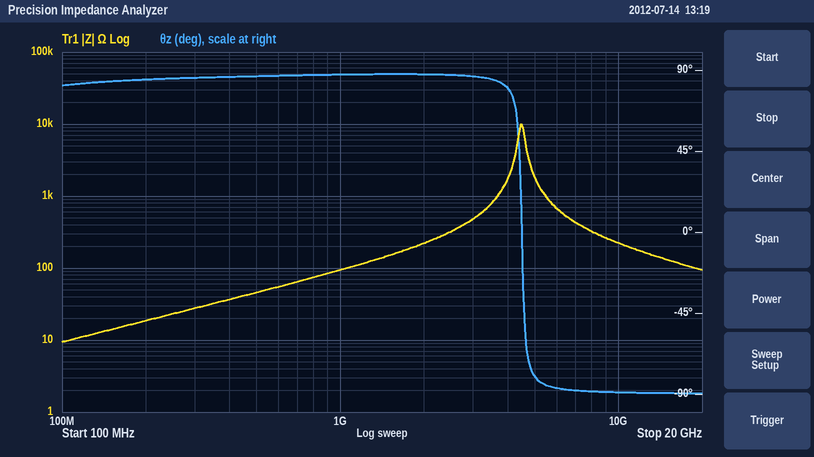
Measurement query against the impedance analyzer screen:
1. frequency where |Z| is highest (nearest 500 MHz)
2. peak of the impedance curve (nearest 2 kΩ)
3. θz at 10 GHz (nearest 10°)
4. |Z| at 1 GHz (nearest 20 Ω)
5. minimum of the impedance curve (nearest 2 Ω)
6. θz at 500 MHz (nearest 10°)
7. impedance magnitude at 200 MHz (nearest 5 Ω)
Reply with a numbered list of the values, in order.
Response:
1. 4.5 GHz
2. 10 kΩ
3. -90°
4. 100 Ω
5. 10 Ω
6. 90°
7. 20 Ω
